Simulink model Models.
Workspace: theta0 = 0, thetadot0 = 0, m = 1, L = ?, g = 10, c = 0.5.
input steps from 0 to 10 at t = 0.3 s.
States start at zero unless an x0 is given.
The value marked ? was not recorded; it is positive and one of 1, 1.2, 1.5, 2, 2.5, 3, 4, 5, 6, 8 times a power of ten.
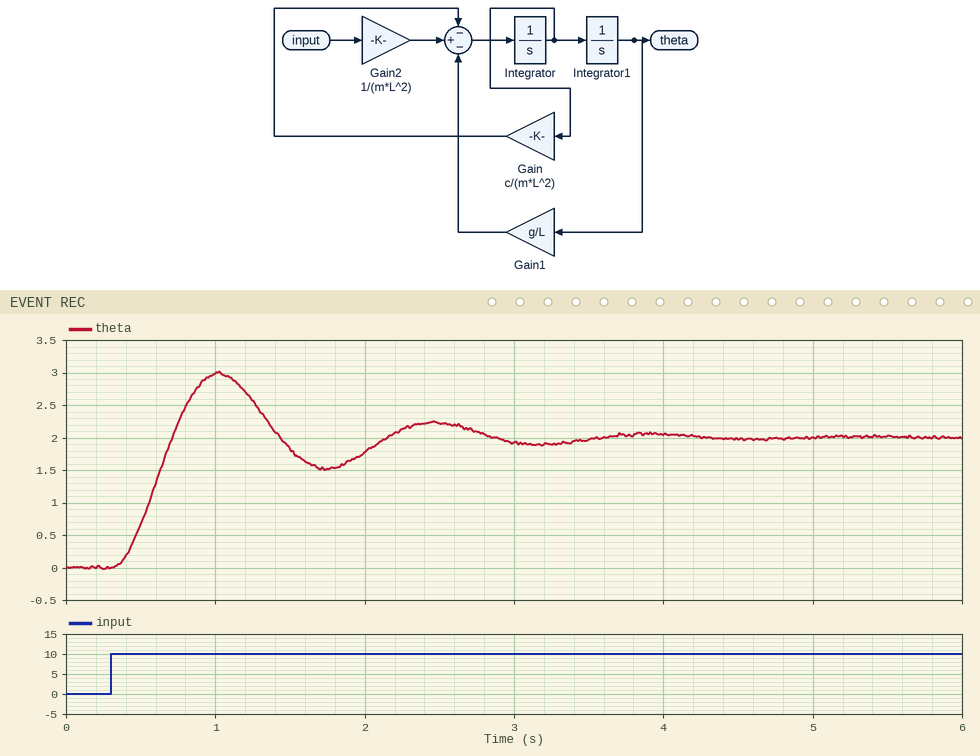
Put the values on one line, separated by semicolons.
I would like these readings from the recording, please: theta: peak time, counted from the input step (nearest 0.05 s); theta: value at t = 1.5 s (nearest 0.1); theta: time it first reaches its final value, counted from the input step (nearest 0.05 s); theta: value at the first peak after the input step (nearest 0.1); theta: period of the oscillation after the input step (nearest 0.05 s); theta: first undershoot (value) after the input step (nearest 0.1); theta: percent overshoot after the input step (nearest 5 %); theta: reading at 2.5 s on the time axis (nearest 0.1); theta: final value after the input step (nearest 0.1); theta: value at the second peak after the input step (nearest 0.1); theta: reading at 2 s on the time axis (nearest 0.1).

0.70 s; 1.8; 0.40 s; 3.0; 1.45 s; 1.5; 50 %; 2.2; 2.0; 2.2; 1.8
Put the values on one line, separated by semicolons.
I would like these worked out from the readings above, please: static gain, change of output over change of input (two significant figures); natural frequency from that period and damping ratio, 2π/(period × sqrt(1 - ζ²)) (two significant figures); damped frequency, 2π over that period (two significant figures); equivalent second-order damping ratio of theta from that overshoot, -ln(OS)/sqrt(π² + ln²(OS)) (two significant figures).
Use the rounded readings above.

0.20; 4.4 rad/s; 4.3 rad/s; 0.22
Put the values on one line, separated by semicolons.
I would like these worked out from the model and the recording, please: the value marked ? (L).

0.5
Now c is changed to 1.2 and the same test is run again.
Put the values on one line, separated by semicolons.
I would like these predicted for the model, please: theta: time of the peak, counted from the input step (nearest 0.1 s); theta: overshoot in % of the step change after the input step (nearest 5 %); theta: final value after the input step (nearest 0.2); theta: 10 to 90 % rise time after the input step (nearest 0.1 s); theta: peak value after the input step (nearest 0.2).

0.8 s; 15 %; 2.0; 0.4 s; 2.2
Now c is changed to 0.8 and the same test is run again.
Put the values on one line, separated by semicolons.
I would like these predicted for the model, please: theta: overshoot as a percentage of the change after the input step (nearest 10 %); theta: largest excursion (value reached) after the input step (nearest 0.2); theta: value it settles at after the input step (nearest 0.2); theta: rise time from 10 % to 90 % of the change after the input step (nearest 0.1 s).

30 %; 2.6; 2.0; 0.3 s
